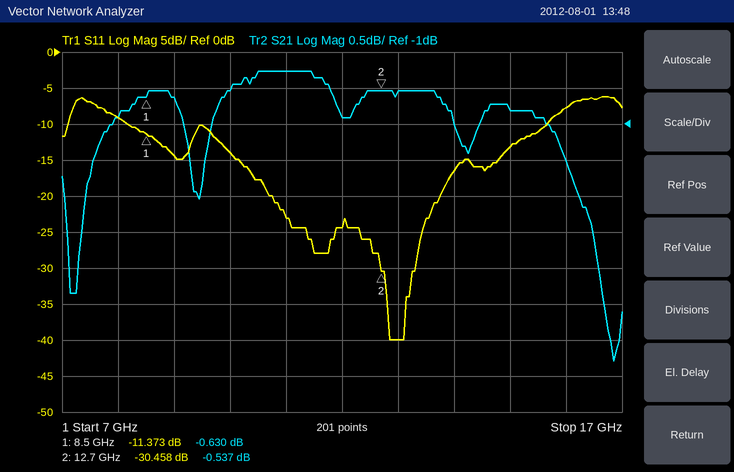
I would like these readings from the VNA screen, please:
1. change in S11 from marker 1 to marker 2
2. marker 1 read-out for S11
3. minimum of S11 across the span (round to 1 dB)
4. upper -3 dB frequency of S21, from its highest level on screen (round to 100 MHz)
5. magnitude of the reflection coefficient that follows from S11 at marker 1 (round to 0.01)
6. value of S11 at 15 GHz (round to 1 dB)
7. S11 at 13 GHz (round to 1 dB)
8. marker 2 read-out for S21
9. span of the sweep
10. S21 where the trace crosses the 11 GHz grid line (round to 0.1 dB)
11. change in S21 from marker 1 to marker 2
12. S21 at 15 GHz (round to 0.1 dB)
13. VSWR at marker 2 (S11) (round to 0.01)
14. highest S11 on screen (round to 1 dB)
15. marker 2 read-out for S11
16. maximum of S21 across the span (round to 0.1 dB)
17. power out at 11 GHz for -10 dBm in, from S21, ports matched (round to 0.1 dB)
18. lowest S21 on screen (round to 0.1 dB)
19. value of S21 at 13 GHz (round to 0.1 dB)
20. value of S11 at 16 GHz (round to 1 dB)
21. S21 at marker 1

-19.085 dB
-11.373 dB
-40 dB
16.6 GHz
0.27
-13 dB
-40 dB
-0.537 dB
10 GHz
-0.3 dB
0.093 dB
-0.8 dB
1.06
-6 dB
-30.458 dB
-0.3 dB
-10.3 dBm
-4.3 dB
-0.5 dB
-8 dB
-0.630 dB
